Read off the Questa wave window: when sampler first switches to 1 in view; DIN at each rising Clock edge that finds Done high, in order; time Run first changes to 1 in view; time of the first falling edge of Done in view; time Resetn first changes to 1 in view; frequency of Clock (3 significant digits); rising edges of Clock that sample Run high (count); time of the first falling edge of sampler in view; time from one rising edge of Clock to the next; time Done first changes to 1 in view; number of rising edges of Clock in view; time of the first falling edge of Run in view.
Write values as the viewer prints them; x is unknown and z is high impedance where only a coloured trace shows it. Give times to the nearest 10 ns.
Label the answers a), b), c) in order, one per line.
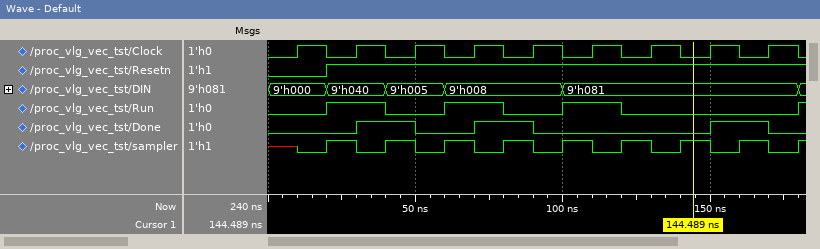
a) 20 ns
b) 9'h005, 9'h008, 9'h081
c) 20 ns
d) 50 ns
e) 20 ns
f) 50.0 MHz
g) 3
h) 30 ns
i) 20 ns
j) 30 ns
k) 9
l) 40 ns
